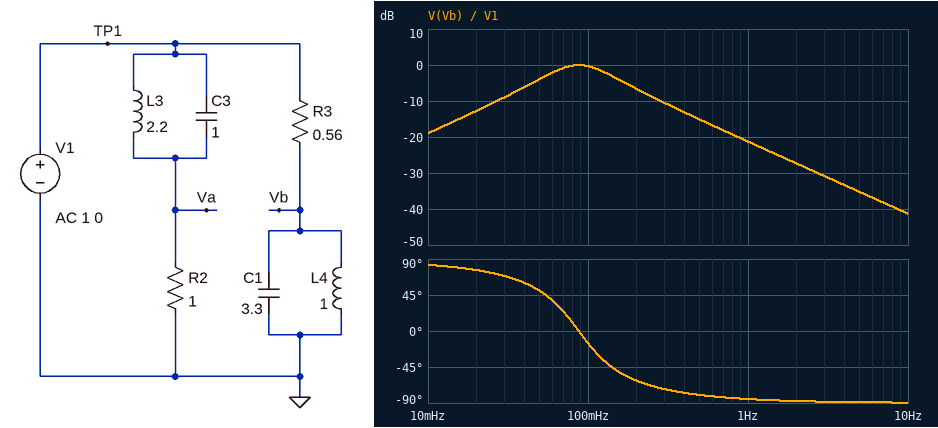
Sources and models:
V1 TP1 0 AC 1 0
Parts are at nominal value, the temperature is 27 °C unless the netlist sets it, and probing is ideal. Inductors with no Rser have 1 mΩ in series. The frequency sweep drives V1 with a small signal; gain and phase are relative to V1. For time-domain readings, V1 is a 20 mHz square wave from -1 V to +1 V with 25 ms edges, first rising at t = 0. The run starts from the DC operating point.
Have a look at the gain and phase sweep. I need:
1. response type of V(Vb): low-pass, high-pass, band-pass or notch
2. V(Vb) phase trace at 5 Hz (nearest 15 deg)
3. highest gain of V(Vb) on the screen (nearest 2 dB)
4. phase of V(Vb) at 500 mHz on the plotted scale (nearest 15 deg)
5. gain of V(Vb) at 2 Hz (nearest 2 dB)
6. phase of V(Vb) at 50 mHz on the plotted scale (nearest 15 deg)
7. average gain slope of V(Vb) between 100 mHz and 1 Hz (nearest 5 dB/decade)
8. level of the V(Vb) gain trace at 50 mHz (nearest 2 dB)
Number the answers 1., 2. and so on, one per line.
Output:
1. band-pass
2. -90 deg
3. 0 dB
4. -75 deg
5. -28 dB
6. 45 deg
7. -20 dB/decade
8. -4 dB
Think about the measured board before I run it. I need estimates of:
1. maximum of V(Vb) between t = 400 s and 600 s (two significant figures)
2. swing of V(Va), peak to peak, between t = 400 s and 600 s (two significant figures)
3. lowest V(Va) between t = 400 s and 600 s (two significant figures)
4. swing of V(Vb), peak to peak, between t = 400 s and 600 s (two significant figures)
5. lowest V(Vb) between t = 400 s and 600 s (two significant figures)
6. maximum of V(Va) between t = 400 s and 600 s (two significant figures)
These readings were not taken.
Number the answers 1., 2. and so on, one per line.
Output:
1. 1.1 V
2. 2.1 V
3. -1.0 V
4. 2.2 V
5. -1.1 V
6. 1.0 V
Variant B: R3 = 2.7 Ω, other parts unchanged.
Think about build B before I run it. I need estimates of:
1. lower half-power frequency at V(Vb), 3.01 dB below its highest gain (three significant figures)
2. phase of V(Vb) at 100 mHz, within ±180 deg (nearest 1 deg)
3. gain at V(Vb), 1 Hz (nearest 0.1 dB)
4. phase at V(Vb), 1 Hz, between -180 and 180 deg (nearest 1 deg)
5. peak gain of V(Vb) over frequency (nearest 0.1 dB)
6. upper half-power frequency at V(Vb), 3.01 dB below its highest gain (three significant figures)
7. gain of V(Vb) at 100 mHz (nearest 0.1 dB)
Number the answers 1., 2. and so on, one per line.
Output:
1. 79.1 mHz
2. -52 deg
3. -34.9 dB
4. -89 deg
5. -0.1 dB
6. 97.1 mHz
7. -4.3 dB
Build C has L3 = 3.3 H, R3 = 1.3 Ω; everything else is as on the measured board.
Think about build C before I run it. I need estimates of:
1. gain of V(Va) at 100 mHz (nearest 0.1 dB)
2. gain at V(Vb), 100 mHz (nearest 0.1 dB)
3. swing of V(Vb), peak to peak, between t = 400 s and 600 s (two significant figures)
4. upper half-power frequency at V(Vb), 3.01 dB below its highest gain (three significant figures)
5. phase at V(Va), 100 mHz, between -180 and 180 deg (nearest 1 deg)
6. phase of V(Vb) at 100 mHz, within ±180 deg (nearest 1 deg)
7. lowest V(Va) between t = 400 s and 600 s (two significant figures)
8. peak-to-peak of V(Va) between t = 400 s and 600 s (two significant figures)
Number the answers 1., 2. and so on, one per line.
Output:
1. -16.8 dB
2. -1.5 dB
3. 1.2 V
4. 108 mHz
5. 82 deg
6. -32 deg
7. -1.0 V
8. 2.0 V
